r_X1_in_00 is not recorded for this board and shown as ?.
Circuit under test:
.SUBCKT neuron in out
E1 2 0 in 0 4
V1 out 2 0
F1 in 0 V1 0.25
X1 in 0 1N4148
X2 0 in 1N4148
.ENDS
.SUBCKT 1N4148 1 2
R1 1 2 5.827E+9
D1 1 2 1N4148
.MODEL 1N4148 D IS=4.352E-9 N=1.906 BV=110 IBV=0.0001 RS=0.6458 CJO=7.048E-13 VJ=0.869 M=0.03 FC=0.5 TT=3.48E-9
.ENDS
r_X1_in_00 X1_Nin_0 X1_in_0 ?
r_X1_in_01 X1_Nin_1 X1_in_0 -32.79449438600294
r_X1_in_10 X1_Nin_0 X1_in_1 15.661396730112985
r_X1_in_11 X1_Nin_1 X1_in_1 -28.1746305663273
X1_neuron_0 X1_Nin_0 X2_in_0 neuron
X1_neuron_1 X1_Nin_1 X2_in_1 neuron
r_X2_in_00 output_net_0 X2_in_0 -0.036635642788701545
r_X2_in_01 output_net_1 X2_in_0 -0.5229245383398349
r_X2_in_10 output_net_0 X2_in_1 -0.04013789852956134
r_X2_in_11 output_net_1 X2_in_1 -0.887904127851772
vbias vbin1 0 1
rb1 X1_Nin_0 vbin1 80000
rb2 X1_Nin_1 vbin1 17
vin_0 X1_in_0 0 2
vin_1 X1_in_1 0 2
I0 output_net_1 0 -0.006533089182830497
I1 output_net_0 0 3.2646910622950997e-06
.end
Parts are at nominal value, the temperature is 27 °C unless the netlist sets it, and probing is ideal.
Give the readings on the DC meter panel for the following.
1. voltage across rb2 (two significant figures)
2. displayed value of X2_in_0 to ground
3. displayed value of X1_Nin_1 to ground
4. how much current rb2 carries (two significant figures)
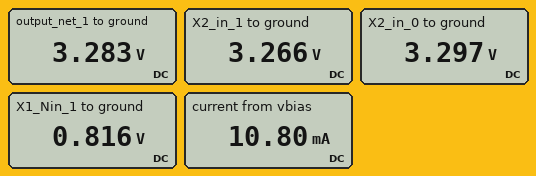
180 mV
3.297 V
0.816 V
11 mA
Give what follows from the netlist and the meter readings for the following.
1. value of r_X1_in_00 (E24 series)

15 Ω
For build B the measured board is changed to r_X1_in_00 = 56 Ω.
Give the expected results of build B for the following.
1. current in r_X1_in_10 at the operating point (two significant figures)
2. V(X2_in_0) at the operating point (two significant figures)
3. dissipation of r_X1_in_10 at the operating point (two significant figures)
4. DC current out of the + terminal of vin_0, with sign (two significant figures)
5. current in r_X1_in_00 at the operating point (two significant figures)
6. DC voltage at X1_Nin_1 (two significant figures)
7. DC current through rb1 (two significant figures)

79 mA
3.0 V
98 mW
-16 mA
22 mA
750 mV
3.0 µA
